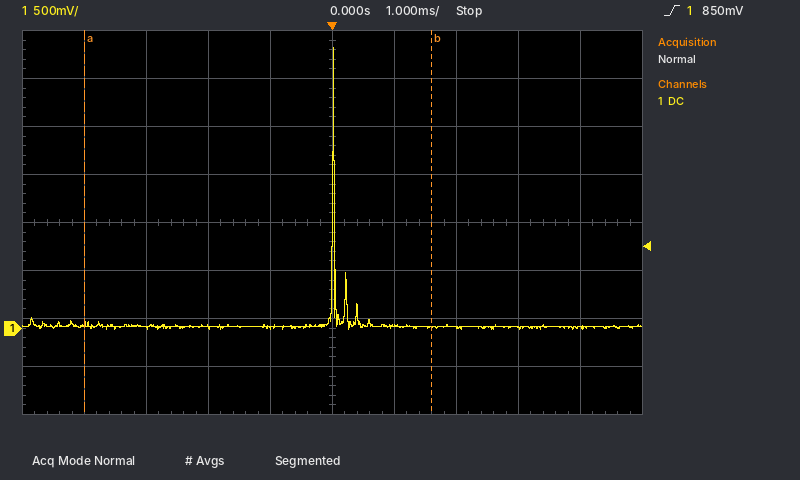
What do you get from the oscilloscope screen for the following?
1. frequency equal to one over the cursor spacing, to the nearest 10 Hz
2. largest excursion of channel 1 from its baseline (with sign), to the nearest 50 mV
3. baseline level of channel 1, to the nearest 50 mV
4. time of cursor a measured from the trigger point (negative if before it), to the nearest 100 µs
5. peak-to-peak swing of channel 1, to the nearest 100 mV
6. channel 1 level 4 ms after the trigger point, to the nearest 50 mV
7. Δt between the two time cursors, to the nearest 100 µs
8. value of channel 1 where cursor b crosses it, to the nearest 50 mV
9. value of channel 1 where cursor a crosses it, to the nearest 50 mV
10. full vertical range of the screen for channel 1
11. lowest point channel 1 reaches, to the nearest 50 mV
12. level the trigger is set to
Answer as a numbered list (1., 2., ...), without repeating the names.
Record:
1. 180 Hz
2. +2.90 V
3. 0 mV
4. -4.0 ms
5. 2.90 V
6. 0 mV
7. 5.6 ms
8. 0 mV
9. 50 mV
10. 4 V
11. 0 mV
12. 850 mV
